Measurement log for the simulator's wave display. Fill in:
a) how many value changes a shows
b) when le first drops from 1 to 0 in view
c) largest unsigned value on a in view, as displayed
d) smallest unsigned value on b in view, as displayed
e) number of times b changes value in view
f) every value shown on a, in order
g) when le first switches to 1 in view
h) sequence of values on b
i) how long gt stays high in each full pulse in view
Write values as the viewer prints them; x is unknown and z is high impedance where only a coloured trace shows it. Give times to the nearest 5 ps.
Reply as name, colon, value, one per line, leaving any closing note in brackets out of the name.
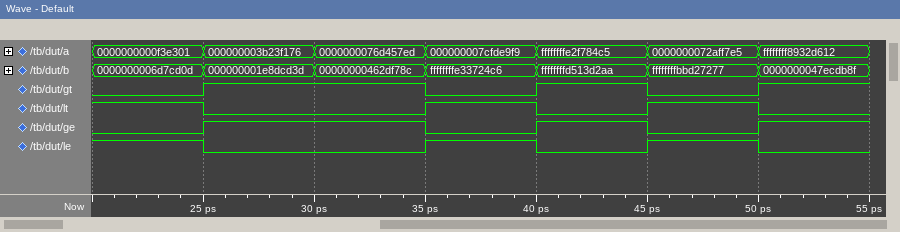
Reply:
how many value changes a shows: 6
when le first drops from 1 to 0 in view: 25 ps
largest unsigned value on a in view, as displayed: ffffffffe2f784c5
smallest unsigned value on b in view, as displayed: 0000000006d7cd0d
number of times b changes value in view: 6
every value shown on a, in order: 0000000000f3e301, 000000003b23f176, 0000000076d457ed, 000000007cfde9f9, ffffffffe2f784c5, 0000000072aff7e5, ffffffff8932d612
when le first switches to 1 in view: 35 ps
sequence of values on b: 0000000006d7cd0d, 000000001e8dcd3d, 00000000462df78c, ffffffffe33724c6, ffffffffd513d2aa, ffffffffbbd27277, 0000000047ecdb8f
how long gt stays high in each full pulse in view: 10 ps, 5 ps
